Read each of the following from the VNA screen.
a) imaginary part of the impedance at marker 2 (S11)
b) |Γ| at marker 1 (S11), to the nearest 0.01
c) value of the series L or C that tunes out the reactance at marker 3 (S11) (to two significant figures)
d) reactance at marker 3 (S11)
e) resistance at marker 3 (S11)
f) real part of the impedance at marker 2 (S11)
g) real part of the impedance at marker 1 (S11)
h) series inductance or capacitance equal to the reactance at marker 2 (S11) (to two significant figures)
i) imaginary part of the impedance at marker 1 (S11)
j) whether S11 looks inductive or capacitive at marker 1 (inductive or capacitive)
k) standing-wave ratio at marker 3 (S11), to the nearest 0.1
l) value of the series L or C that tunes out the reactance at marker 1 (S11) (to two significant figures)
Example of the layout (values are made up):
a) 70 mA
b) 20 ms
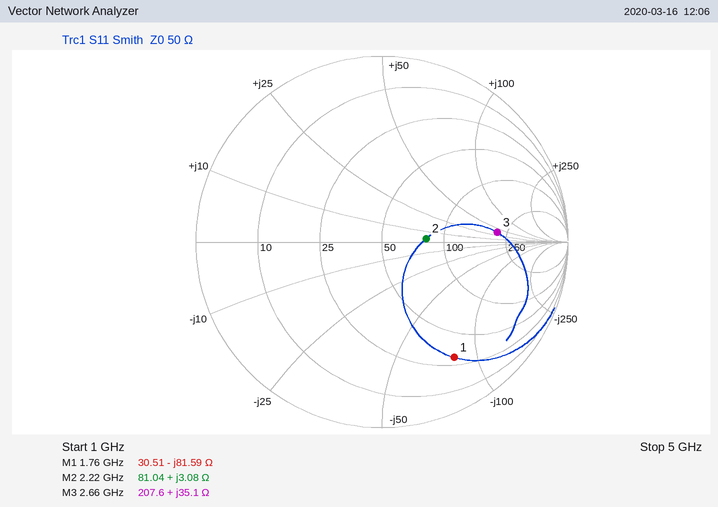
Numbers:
a) +3.08 Ω
b) 0.73
c) 1.7 pF
d) +35.1 Ω
e) 207.6 Ω
f) 81.04 Ω
g) 30.51 Ω
h) 220 pH
i) -81.59 Ω
j) capacitive
k) 4.3
l) 7.4 nH
